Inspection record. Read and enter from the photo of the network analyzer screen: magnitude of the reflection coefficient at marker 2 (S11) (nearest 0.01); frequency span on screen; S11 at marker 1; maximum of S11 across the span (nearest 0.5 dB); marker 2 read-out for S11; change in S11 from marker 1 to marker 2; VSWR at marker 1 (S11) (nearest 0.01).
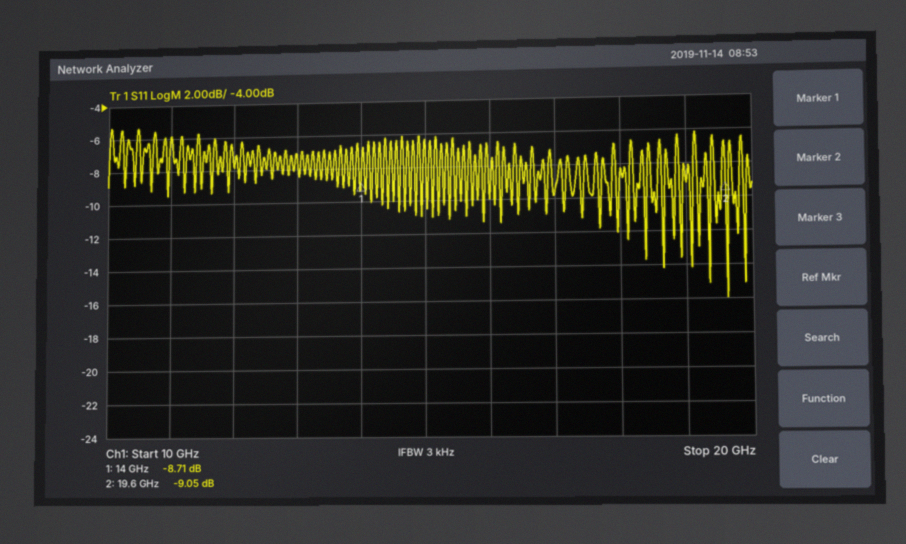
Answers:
0.35
10 GHz
-8.71 dB
-5.5 dB
-9.05 dB
-0.34 dB
2.16
